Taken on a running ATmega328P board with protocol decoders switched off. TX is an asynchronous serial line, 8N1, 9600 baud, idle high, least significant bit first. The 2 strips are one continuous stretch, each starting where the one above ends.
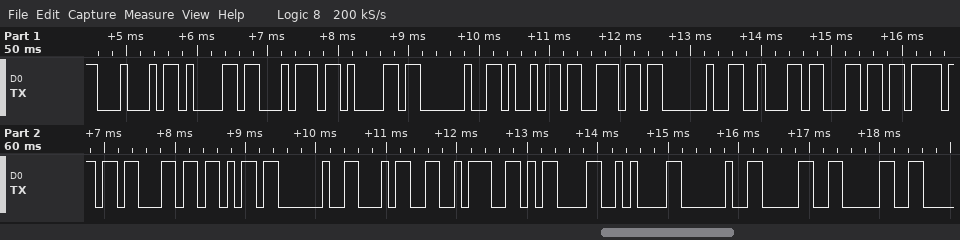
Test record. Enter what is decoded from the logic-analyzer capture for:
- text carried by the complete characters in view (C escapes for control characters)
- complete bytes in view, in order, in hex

"Data in block 4:\r\n 00"
44 61 74 61 20 69 6E 20 62 6C 6F 63 6B 20 34 3A 0D 0A 20 30 30
